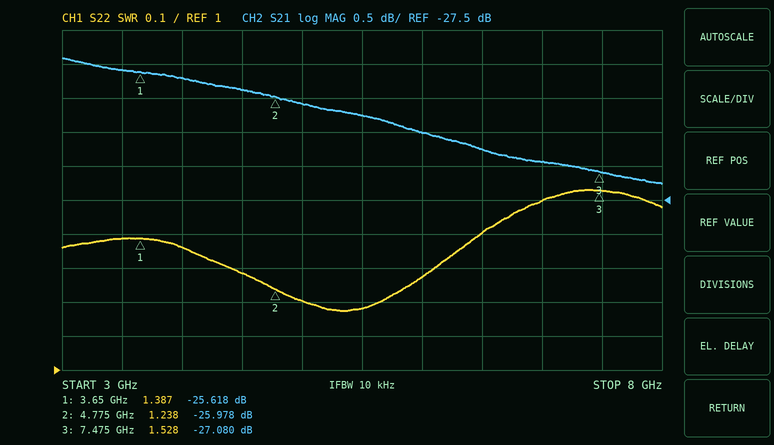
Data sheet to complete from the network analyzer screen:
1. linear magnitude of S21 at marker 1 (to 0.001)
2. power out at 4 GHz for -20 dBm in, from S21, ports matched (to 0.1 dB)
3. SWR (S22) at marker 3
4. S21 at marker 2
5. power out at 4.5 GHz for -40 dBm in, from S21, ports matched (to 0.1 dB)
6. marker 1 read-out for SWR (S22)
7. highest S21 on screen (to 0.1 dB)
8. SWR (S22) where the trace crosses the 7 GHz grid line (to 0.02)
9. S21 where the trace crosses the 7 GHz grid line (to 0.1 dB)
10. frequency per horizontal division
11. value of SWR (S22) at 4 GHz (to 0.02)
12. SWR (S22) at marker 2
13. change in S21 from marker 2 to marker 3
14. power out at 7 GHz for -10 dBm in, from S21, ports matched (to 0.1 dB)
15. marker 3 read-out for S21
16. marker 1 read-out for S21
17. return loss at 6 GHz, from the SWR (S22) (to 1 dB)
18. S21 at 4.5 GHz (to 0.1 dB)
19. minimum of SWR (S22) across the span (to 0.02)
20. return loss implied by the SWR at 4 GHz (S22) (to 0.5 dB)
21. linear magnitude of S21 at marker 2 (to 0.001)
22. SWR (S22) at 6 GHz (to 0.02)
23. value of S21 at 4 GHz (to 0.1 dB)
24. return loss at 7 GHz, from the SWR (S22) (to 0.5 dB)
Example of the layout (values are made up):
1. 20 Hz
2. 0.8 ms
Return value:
1. 0.052
2. -45.7 dBm
3. 1.528
4. -25.978 dB
5. -65.9 dBm
6. 1.387
7. -25.4 dB
8. 1.50
9. -26.9 dB
10. 500 MHz
11. 1.36
12. 1.238
13. -1.102 dB
14. -36.9 dBm
15. -27.080 dB
16. -25.618 dB
17. 18 dB
18. -25.9 dB
19. 1.18
20. 16.5 dB
21. 0.050
22. 1.28
23. -25.7 dB
24. 14.0 dB
